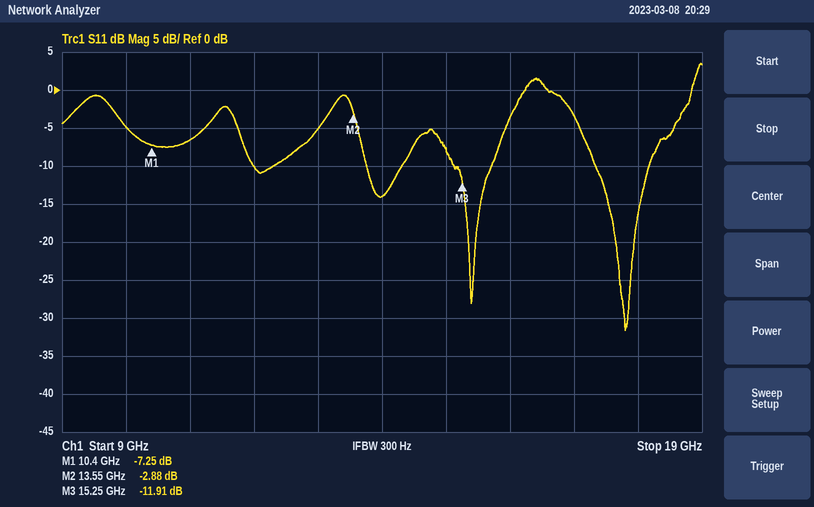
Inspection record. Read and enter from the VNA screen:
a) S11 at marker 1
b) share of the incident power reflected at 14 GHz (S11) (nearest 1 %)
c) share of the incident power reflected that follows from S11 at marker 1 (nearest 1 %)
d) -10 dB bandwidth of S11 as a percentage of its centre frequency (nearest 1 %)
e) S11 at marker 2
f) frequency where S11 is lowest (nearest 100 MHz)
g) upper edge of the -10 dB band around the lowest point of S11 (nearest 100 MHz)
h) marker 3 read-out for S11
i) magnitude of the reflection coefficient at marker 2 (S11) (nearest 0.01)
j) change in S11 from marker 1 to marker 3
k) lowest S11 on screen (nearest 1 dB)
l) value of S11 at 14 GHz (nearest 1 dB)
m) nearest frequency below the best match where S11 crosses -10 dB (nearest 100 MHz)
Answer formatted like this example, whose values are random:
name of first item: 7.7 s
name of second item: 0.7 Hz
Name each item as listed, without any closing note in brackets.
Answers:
S11 at marker 1: -7.25 dB
share of the incident power reflected at 14 GHz (S11): 4 %
share of the incident power reflected that follows from S11 at marker 1: 19 %
-10 dB bandwidth of S11 as a percentage of its centre frequency: 5 %
S11 at marker 2: -2.88 dB
frequency where S11 is lowest: 17.8 GHz
upper edge of the -10 dB band around the lowest point of S11: 18.2 GHz
marker 3 read-out for S11: -11.91 dB
magnitude of the reflection coefficient at marker 2 (S11): 0.72
change in S11 from marker 1 to marker 3: -4.66 dB
lowest S11 on screen: -32 dB
value of S11 at 14 GHz: -14 dB
nearest frequency below the best match where S11 crosses -10 dB: 17.3 GHz
